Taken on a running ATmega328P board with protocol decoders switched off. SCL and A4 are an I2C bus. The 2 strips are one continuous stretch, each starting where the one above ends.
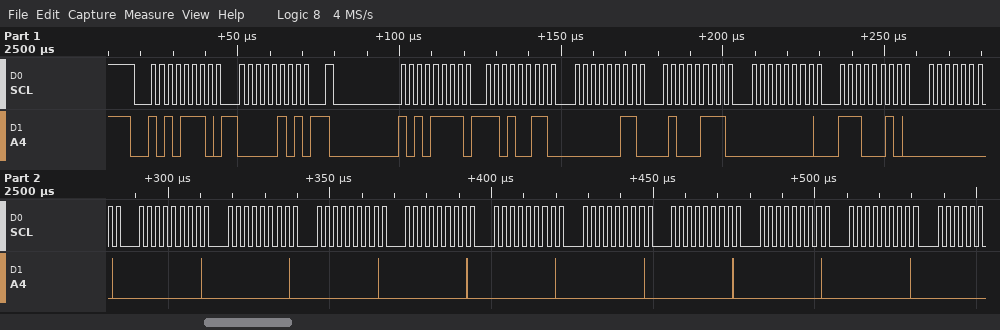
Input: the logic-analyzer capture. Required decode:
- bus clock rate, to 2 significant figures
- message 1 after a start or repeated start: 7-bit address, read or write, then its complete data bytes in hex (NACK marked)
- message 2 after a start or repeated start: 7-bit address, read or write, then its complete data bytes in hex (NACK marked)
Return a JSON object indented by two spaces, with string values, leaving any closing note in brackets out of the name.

{
  "bus clock rate, to 2 significant figures": "400 kHz",
  "message 1 after a start or repeated start: 7-bit address, read or write, then its complete data bytes in hex": "0x57 write: 05",
  "message 2 after a start or repeated start: 7-bit address, read or write, then its complete data bytes in hex": "0x57 read: D3 03 47 00 E2 00 00 00 00 00 00 00 00 00 00"
}
